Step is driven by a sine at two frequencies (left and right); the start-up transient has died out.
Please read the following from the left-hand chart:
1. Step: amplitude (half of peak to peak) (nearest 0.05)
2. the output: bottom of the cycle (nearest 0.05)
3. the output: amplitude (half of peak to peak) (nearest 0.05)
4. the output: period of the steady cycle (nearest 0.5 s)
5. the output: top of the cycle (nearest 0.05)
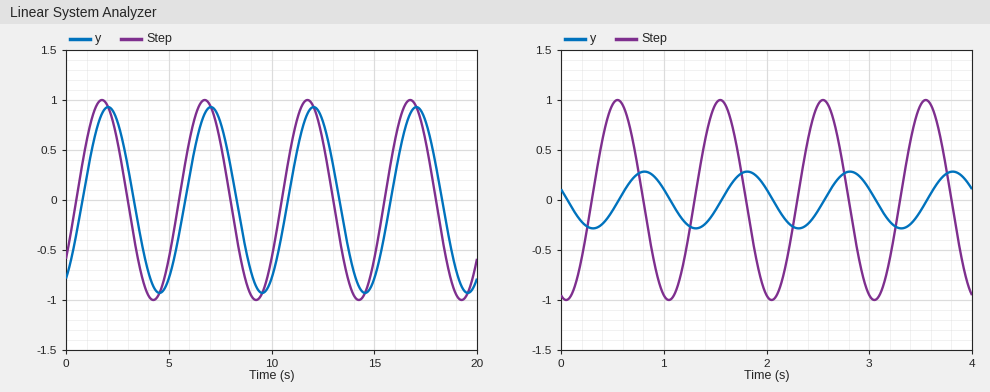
1.00
-0.95
0.95
5.0 s
0.95
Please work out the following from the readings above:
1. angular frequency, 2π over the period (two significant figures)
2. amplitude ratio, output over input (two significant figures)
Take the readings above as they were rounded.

1.3 rad/s
0.95
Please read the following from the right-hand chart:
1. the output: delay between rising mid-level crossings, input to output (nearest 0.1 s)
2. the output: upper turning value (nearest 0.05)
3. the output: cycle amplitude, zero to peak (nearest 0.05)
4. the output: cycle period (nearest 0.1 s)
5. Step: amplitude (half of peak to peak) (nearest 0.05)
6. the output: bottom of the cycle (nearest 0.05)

0.3 s
0.30
0.30
1.0 s
1.00
-0.30
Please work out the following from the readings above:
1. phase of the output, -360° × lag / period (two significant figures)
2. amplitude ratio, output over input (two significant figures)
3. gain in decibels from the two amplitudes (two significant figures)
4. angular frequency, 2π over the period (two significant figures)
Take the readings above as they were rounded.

-110°
0.30
-10 dB
6.3 rad/s
